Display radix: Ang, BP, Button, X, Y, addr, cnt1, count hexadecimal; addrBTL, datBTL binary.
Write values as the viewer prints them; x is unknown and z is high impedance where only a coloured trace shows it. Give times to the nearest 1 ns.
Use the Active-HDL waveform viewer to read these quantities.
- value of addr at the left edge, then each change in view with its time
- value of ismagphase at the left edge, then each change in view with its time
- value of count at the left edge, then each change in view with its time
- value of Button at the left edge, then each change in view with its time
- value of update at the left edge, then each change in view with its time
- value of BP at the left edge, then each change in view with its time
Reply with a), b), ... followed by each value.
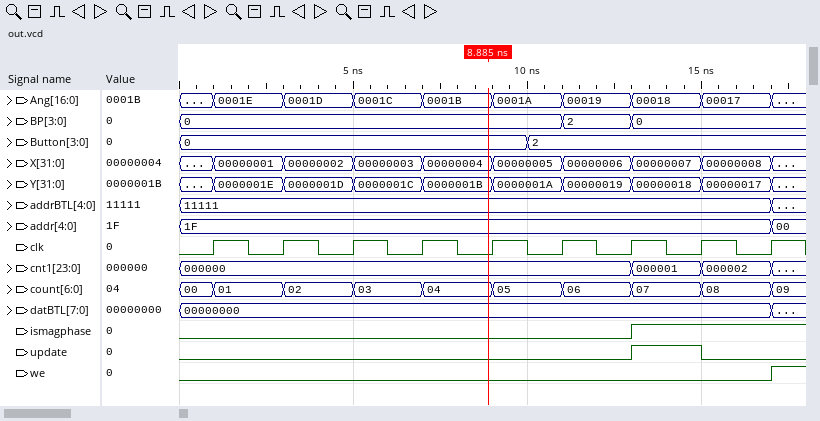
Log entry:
a) 1F, 00 at 17 ns
b) 0, 1 at 13 ns
c) 00, 01 at 1 ns, 02 at 3 ns, 03 at 5 ns, 04 at 7 ns, 05 at 9 ns, 06 at 11 ns, 07 at 13 ns, 08 at 15 ns, 09 at 17 ns
d) 0, 2 at 10 ns
e) 0, 1 at 13 ns, 0 at 15 ns
f) 0, 2 at 11 ns, 0 at 13 ns
